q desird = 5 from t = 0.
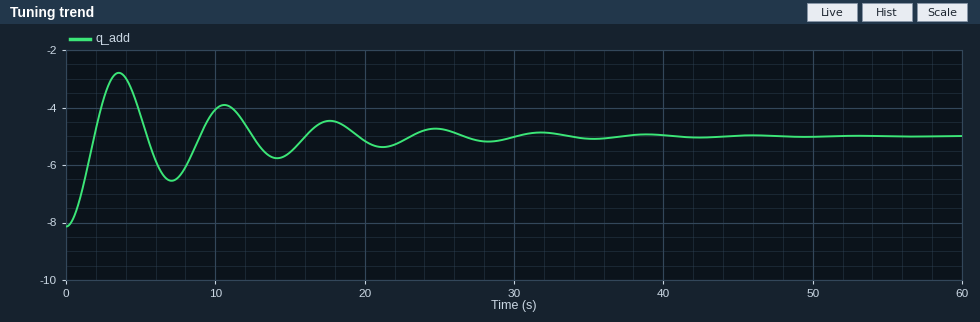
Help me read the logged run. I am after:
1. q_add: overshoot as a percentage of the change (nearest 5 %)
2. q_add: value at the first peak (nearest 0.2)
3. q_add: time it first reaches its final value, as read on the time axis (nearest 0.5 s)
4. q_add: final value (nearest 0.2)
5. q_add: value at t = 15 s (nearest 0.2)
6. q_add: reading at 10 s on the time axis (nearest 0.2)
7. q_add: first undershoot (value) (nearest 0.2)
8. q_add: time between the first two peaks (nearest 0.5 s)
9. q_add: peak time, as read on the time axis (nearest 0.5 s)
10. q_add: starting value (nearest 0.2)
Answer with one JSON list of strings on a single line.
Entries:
["70 %", "-2.8", "2.0 s", "-5.0", "-5.6", "-4.0", "-6.6", "7.0 s", "3.5 s", "-8.2"]
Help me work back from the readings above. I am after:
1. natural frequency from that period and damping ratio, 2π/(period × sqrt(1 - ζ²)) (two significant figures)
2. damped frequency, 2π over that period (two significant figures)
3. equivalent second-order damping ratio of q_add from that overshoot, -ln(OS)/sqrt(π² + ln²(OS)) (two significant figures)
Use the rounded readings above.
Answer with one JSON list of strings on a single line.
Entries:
["0.90 rad/s", "0.90 rad/s", "0.11"]
